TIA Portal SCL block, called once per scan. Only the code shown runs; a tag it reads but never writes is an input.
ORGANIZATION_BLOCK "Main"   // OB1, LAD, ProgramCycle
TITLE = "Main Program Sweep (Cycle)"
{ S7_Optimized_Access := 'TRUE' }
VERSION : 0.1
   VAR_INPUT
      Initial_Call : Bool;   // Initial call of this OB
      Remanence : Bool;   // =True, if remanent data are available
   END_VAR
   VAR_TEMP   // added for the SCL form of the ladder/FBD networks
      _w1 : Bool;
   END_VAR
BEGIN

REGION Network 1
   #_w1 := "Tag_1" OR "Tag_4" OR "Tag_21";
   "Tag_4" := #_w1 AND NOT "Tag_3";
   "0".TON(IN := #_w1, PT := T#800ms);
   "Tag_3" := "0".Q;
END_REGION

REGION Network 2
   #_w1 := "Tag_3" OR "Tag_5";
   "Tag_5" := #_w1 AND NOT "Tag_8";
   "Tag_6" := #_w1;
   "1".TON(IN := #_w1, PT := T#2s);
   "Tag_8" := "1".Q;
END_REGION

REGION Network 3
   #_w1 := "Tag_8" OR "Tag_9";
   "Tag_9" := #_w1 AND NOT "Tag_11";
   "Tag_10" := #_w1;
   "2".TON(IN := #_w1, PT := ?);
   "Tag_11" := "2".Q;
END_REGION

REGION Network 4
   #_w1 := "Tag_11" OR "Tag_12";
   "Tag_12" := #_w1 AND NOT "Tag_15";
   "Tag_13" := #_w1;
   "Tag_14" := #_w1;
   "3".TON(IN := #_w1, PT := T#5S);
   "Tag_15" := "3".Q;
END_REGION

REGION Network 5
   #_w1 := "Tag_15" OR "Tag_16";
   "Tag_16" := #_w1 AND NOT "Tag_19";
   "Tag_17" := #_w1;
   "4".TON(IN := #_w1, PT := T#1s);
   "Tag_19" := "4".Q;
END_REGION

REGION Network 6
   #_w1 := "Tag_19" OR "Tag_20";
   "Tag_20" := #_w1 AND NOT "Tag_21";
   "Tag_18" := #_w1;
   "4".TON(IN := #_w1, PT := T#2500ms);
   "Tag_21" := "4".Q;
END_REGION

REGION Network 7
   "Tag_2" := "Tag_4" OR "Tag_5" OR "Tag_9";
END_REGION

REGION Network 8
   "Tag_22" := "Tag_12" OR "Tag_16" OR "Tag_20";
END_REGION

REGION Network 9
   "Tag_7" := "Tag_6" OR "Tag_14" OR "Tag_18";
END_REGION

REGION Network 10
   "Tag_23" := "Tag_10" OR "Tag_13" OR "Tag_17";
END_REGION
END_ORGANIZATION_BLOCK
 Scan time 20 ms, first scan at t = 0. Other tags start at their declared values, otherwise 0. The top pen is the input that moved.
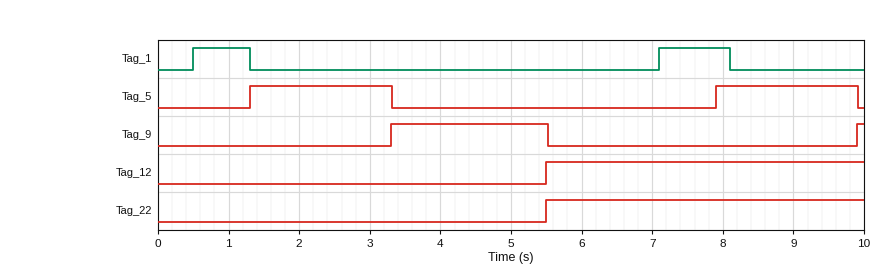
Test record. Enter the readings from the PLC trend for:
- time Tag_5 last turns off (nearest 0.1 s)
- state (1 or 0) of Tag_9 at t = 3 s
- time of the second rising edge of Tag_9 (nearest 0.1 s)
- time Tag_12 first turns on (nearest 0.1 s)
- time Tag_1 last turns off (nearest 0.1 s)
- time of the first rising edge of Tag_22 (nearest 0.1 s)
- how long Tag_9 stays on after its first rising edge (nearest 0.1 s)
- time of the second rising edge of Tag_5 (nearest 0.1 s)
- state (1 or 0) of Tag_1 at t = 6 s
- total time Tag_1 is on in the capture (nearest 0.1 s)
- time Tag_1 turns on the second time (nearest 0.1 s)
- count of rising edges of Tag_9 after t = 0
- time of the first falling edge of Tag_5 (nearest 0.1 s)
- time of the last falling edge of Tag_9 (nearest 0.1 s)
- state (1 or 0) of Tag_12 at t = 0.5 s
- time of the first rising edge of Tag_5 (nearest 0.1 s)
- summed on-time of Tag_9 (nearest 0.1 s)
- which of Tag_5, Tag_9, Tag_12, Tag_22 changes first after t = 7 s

9.9 s
0
9.9 s
5.5 s
8.1 s
5.5 s
2.2 s
7.9 s
0
1.8 s
7.1 s
2
3.3 s
5.5 s
0
1.3 s
2.3 s
Tag_5
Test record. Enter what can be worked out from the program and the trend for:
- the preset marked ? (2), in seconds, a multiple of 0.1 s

2.2 s
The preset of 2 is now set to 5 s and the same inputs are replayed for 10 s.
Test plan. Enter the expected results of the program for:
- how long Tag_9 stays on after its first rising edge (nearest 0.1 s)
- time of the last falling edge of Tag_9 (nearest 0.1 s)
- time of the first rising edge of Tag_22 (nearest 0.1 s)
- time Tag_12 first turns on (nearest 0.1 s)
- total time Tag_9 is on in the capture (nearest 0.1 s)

5.0 s
8.3 s
8.3 s
8.3 s
5.1 s
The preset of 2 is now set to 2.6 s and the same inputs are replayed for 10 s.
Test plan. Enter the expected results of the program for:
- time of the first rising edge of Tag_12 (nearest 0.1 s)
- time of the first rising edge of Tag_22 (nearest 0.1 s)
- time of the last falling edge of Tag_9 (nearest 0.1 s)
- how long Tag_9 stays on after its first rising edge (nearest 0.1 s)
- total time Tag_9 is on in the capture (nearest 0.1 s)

5.9 s
5.9 s
5.9 s
2.6 s
2.7 s
